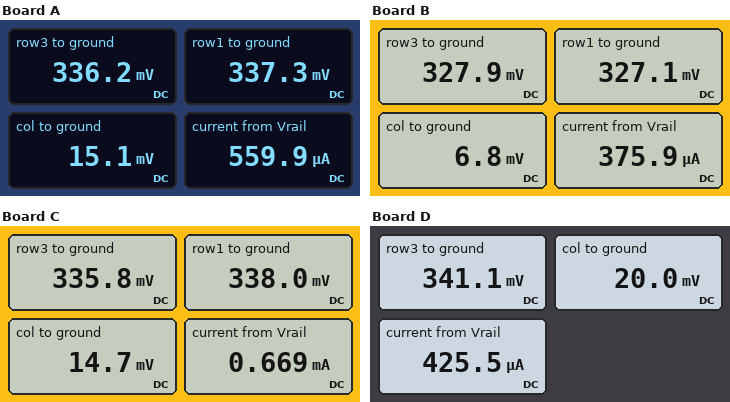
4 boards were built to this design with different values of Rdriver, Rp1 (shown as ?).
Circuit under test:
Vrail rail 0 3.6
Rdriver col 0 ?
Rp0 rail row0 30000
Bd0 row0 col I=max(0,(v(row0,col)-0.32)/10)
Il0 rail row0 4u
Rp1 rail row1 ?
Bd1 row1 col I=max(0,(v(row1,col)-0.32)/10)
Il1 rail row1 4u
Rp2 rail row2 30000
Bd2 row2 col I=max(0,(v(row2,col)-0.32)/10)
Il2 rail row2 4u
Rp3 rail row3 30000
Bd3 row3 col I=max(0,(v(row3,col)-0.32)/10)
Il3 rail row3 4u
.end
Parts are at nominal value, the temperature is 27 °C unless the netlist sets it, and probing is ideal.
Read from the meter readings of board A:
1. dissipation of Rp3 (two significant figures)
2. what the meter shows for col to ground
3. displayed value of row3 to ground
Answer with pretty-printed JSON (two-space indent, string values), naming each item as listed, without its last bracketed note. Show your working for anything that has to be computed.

{
  "dissipation of Rp3": "(3.6 V - 336.2 mV)^2 / 30 kΩ = 360 µW",
  "what the meter shows for col to ground": "15.1 mV",
  "displayed value of row3 to ground": "336.2 mV"
}
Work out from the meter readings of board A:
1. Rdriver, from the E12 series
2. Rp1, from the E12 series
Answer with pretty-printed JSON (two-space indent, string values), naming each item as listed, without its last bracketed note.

{
  "Rdriver, from the E12 series": "27 Ω",
  "Rp1, from the E12 series": "15 kΩ"
}
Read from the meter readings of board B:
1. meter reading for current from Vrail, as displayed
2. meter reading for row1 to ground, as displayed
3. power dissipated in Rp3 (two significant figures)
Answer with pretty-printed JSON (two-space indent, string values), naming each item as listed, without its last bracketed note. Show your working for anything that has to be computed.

{
  "meter reading for current from Vrail, as displayed": "375.9 µA",
  "meter reading for row1 to ground, as displayed": "327.1 mV",
  "power dissipated in Rp3": "(3.6 V - 327.9 mV)^2 / 30 kΩ = 360 µW"
}
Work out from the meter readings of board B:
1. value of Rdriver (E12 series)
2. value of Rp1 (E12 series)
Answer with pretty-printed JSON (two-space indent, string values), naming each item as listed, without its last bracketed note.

{
  "value of Rdriver": "18 Ω",
  "value of Rp1": "100 kΩ"
}
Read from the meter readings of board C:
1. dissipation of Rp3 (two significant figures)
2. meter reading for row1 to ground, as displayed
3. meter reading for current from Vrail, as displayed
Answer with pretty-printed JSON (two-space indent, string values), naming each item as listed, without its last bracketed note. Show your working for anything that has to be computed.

{
  "dissipation of Rp3": "(3.6 V - 335.8 mV)^2 / 30 kΩ = 360 µW",
  "meter reading for row1 to ground, as displayed": "338.0 mV",
  "meter reading for current from Vrail, as displayed": "0.669 mA"
}
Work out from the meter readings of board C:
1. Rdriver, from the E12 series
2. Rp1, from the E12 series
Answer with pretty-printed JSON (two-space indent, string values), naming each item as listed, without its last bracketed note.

{
  "Rdriver, from the E12 series": "22 Ω",
  "Rp1, from the E12 series": "10 kΩ"
}
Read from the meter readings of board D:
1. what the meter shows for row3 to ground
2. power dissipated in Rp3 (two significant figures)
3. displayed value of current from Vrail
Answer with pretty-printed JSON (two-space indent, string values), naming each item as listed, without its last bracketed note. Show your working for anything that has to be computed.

{
  "what the meter shows for row3 to ground": "341.1 mV",
  "power dissipated in Rp3": "(3.6 V - 341.1 mV)^2 / 30 kΩ = 350 µW",
  "displayed value of current from Vrail": "425.5 µA"
}
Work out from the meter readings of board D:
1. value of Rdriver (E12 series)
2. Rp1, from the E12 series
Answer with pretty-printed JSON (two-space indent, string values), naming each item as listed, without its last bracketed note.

{
  "value of Rdriver": "47 Ω",
  "Rp1, from the E12 series": "39 kΩ"
}
